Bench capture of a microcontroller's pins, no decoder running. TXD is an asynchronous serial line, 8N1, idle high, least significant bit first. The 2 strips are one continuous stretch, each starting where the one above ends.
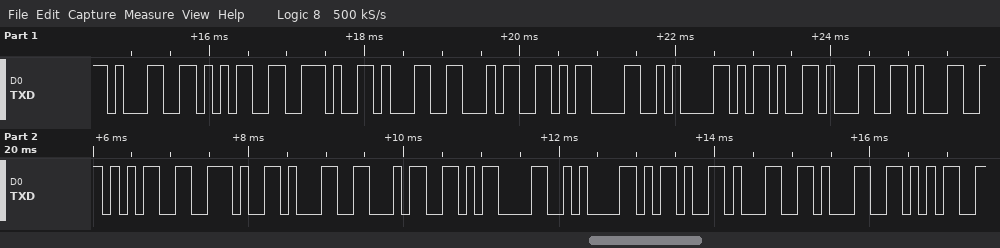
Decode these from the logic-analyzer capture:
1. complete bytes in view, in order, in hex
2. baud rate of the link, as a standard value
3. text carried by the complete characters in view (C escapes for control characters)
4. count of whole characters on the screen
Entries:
0x31 0x35 0x2E 0x31 0x34 0x0D 0x0A 0x2D 0x31 0x31 0x35 0x2E 0x31 0x34 0x0D 0x0A 0x2D 0x31 0x31 0x35
9600 baud
"15.14\r\n-115.14\r\n-115"
20
